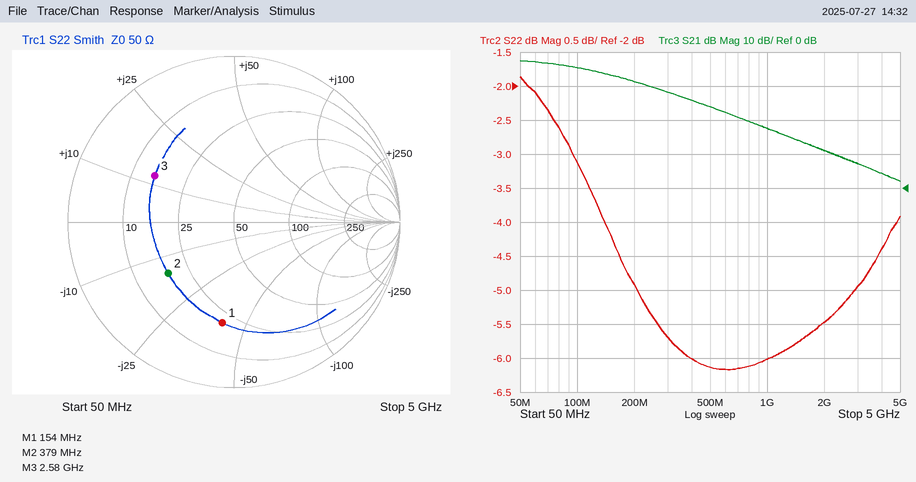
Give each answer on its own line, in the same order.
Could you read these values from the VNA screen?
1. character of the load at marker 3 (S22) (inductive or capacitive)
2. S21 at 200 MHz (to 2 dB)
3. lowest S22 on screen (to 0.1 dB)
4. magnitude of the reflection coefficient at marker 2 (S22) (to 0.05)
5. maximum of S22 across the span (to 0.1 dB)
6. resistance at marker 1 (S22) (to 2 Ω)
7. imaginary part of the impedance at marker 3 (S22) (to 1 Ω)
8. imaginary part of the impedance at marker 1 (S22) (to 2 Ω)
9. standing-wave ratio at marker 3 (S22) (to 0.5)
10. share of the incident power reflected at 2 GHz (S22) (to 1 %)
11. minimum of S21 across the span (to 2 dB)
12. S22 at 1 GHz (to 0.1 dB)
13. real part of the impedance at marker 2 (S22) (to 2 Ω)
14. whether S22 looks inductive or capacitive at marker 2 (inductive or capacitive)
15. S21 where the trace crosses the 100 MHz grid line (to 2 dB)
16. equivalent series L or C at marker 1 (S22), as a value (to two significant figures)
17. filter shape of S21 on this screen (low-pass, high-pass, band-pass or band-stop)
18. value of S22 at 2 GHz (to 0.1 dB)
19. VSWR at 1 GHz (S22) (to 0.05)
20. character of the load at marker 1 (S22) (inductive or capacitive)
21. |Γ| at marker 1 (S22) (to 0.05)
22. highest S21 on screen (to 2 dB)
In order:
inductive
32 dB
-6.2 dB
0.50
-1.9 dB
20 Ω
+12 Ω
-40 Ω
3.5
28 %
2 dB
-6.0 dB
18 Ω
capacitive
36 dB
26 pF
low-pass
-5.5 dB
3.00
capacitive
0.60
38 dB
